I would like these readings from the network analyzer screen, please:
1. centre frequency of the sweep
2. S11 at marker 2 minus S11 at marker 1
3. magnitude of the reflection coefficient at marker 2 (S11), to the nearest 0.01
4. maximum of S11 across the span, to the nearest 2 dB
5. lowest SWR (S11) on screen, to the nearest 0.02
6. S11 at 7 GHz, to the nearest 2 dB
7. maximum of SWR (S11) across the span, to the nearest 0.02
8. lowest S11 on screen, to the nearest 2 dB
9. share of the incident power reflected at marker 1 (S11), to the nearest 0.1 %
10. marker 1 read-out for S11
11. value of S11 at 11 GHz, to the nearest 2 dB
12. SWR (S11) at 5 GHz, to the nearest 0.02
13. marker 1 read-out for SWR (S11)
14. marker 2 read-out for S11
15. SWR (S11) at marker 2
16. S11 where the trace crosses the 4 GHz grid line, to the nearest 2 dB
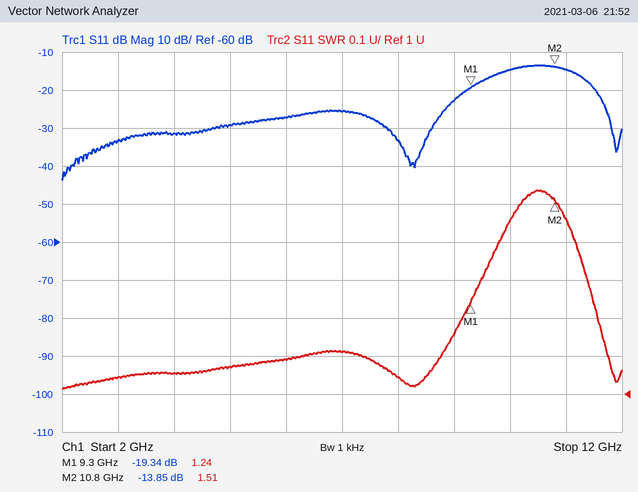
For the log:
7 GHz
5.49 dB
0.20
-14 dB
1.02
-26 dB
1.54
-44 dB
1.2 %
-19.34 dB
-14 dB
1.08
1.24
-13.85 dB
1.51
-32 dB
